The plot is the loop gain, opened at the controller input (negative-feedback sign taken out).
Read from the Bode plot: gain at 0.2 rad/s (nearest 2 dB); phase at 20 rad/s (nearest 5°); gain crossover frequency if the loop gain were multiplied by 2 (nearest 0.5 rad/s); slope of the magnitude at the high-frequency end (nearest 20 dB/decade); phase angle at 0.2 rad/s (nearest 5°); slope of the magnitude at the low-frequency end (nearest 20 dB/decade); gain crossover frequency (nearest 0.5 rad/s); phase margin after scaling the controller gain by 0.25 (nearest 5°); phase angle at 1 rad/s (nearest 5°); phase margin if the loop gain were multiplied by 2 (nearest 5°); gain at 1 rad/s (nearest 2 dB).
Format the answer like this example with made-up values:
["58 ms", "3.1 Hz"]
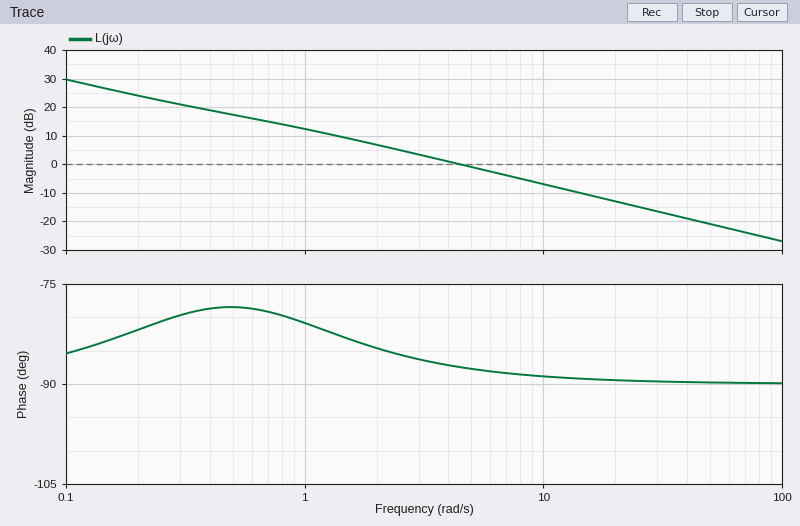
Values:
["24 dB", "-90°", "9.0 rad/s", "-20 dB/decade", "-80°", "-20 dB/decade", "4.5 rad/s", "100°", "-80°", "90°", "12 dB"]
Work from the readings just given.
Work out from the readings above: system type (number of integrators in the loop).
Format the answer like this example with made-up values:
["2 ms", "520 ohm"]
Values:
["1"]
